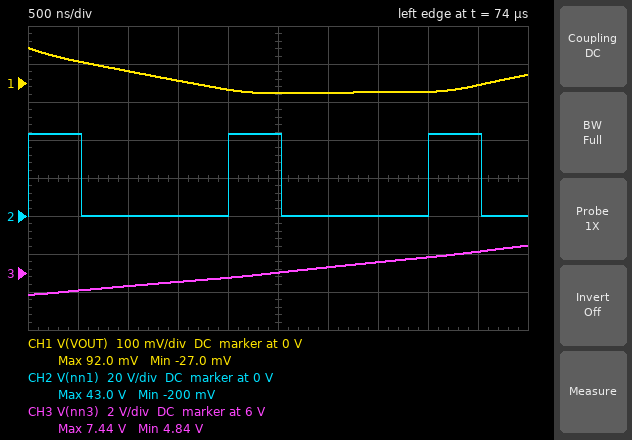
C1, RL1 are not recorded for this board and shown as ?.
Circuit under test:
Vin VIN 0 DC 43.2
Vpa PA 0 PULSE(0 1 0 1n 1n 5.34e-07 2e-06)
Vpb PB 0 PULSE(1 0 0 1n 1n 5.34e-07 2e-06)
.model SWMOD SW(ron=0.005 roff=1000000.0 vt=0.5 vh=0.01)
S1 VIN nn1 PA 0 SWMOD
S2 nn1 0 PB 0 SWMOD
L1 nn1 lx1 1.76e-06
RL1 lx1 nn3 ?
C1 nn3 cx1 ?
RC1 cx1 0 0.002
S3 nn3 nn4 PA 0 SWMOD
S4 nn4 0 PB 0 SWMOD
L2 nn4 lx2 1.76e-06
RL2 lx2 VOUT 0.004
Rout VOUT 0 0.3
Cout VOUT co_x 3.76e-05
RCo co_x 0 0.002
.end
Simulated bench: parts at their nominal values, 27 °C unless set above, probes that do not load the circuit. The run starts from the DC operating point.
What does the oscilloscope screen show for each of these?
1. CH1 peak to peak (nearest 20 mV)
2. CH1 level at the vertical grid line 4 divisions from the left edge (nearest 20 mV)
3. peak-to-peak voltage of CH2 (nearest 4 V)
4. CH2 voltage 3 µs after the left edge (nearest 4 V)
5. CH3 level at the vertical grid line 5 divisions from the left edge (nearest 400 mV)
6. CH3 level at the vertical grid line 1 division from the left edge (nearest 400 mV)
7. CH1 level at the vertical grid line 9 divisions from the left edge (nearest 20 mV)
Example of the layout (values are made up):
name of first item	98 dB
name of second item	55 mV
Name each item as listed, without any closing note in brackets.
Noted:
CH1 peak to peak	120 mV
CH1 level at the vertical grid line 4 divisions from the left edge	-20 mV
peak-to-peak voltage of CH2	44 V
CH2 voltage 3 µs after the left edge	0 V
CH3 level at the vertical grid line 5 divisions from the left edge	6.0 V
CH3 level at the vertical grid line 1 division from the left edge	5.2 V
CH1 level at the vertical grid line 9 divisions from the left edge	0 V
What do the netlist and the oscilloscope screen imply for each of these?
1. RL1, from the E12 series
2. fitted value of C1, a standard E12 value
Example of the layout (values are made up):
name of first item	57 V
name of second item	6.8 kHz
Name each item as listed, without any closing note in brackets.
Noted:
RL1, from the E12 series	1.2 mΩ
fitted value of C1, a standard E12 value	68 µF
